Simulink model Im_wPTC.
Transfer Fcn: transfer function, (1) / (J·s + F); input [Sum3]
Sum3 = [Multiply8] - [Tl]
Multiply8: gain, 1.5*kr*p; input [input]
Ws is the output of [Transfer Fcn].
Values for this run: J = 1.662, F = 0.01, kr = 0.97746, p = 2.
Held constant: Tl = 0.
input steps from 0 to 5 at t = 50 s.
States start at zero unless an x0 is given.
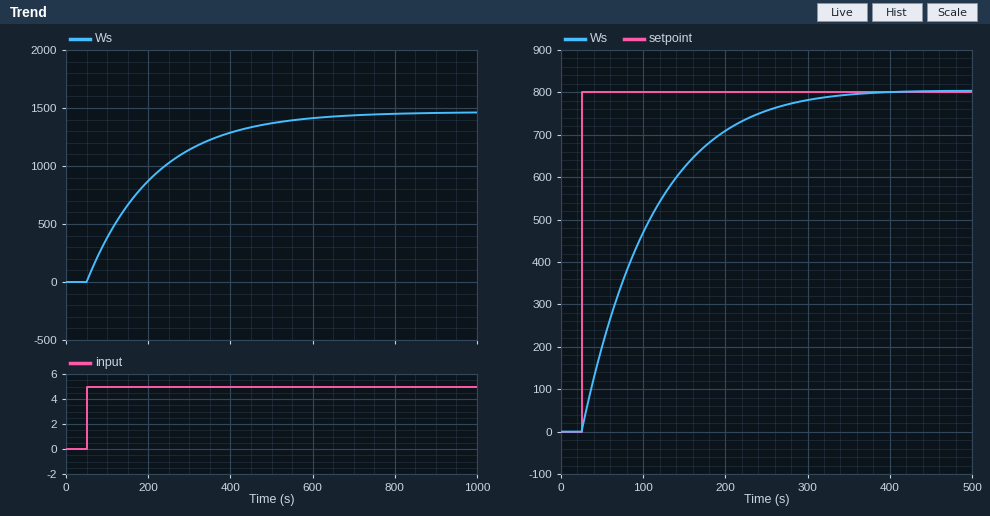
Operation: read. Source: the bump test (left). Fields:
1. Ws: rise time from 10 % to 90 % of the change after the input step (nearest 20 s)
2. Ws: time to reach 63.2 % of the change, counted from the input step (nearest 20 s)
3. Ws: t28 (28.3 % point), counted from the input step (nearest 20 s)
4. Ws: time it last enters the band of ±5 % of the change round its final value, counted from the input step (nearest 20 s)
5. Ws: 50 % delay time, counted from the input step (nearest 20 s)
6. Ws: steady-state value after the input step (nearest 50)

360 s
160 s
60 s
500 s
120 s
1450
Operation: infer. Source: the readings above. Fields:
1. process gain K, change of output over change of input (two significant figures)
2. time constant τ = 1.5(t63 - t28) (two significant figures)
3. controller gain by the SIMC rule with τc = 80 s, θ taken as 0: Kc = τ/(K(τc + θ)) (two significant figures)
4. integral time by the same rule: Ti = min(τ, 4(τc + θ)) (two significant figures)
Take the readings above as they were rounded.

290
150 s
0.0065
150 s
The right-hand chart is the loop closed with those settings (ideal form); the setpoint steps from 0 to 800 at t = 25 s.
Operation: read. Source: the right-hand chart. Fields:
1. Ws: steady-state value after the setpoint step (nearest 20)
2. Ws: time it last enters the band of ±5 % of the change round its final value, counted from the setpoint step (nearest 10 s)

800
230 s
